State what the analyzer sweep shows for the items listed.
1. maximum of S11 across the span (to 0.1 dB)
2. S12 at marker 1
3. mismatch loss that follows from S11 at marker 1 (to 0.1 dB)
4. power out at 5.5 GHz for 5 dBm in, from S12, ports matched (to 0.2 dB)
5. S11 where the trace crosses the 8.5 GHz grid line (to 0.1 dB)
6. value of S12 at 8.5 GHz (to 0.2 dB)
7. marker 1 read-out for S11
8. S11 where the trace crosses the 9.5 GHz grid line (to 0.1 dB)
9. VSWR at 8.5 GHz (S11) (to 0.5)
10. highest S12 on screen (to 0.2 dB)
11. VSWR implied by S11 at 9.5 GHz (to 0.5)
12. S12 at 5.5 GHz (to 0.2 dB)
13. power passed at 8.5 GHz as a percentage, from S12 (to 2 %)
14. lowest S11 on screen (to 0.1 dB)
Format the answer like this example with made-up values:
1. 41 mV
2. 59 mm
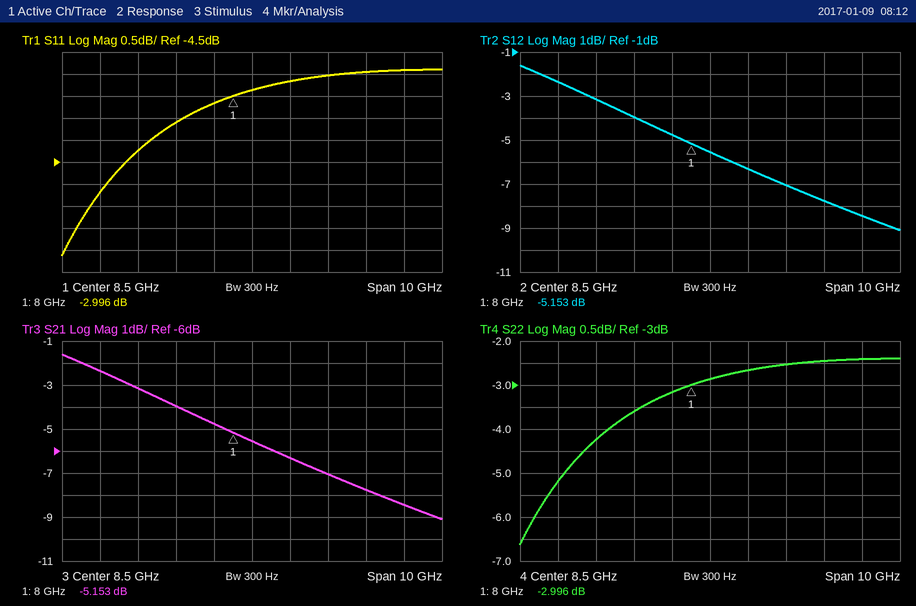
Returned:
1. -2.4 dB
2. -5.153 dB
3. 3.0 dB
4. 1.8 dBm
5. -2.9 dB
6. -5.6 dB
7. -2.996 dB
8. -2.7 dB
9. 6.0
10. -1.6 dB
11. 6.5
12. -3.2 dB
13. 28 %
14. -6.6 dB
